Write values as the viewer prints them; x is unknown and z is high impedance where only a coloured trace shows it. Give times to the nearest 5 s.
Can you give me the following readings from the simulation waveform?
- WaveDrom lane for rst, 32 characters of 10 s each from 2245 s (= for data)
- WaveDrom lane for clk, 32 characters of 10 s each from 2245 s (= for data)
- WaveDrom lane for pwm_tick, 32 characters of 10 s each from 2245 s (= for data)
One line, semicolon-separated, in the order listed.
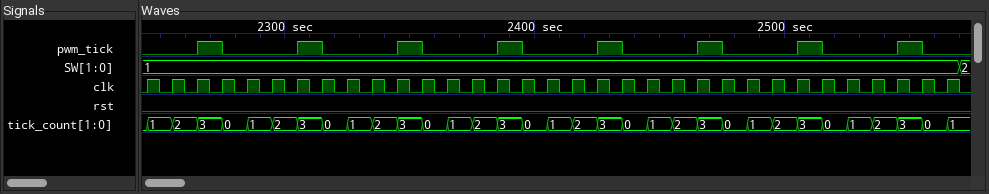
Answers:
{name: 'rst', wave: '0...............................'}; {name: 'clk', wave: 'p...............................'}; {name: 'pwm_tick', wave: '0.10..10..10..10..10..10..10..10'}
